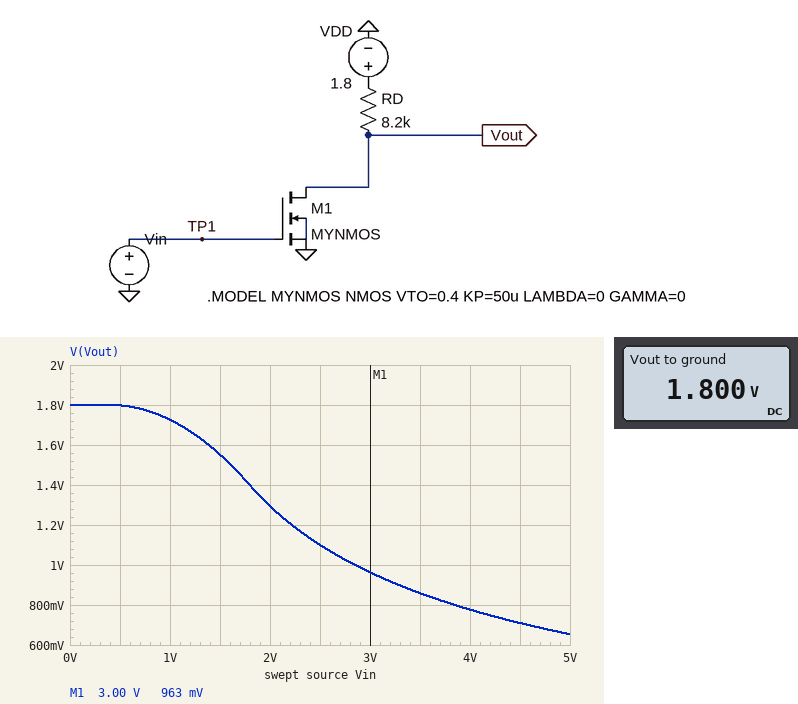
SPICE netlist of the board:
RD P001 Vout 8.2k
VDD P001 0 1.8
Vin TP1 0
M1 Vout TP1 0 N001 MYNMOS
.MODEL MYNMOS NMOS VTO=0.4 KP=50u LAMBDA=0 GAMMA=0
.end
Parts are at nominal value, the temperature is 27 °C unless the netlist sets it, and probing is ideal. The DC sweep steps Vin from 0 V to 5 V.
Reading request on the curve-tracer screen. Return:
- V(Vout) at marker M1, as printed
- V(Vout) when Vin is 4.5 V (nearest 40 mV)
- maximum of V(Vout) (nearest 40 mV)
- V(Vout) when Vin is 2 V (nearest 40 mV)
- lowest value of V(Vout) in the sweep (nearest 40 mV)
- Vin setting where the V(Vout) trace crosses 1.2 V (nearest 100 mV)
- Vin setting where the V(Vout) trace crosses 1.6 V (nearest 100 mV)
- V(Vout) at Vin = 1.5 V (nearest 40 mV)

963 mV
720 mV
1.80 V
1.28 V
640 mV
2.2 V
1.4 V
1.56 V
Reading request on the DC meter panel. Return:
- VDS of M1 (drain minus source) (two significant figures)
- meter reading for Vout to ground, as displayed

1.8 V
1.800 V
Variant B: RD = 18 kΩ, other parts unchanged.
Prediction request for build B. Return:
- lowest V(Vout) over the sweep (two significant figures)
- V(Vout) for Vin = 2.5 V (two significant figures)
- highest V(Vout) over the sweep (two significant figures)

360 mV
700 mV
1.8 V
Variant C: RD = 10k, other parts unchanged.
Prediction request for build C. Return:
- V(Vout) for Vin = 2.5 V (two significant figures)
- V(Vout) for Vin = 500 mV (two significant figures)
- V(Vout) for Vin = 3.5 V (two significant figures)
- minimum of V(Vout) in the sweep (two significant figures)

1.0 V
1.8 V
760 mV
570 mV
